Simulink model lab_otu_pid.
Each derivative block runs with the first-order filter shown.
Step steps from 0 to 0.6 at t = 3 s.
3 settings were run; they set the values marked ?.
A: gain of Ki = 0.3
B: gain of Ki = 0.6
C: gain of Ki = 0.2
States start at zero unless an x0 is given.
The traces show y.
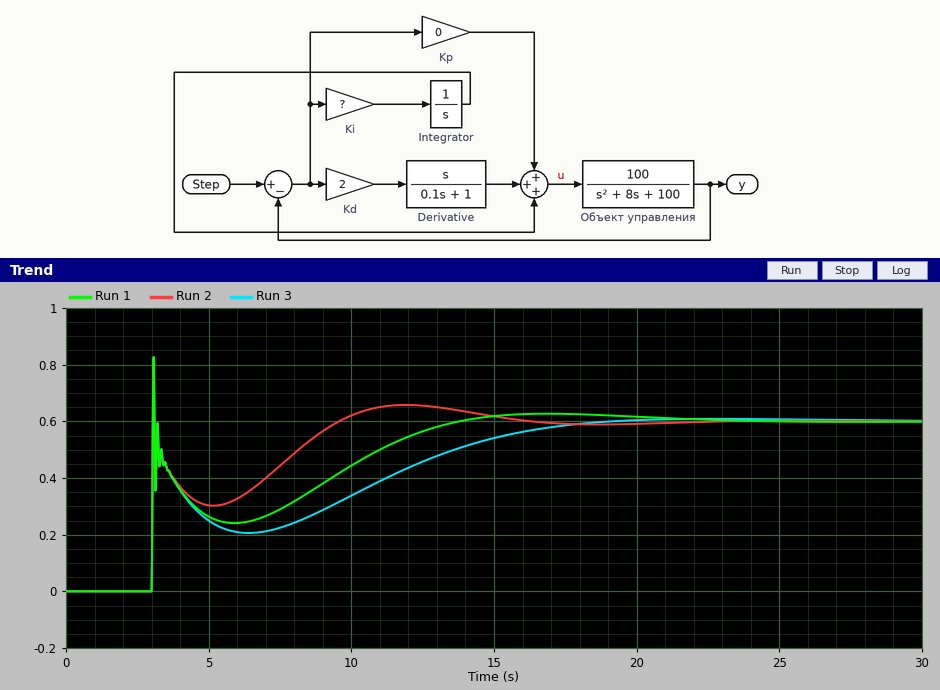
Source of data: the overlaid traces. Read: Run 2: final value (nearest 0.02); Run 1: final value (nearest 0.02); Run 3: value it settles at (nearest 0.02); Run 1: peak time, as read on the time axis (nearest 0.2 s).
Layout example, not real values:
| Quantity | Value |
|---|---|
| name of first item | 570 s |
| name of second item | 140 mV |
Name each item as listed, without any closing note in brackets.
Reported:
| Quantity | Value |
|---|---|
| Run 2: final value | 0.60 |
| Run 1: final value | 0.60 |
| Run 3: value it settles at | 0.60 |
| Run 1: peak time, as read on the time axis | 3.0 s |
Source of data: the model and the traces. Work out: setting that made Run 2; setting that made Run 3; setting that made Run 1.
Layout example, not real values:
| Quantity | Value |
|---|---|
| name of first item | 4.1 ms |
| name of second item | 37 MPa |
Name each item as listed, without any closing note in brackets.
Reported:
| Quantity | Value |
|---|---|
| setting that made Run 2 | B |
| setting that made Run 3 | C |
| setting that made Run 1 | A |
